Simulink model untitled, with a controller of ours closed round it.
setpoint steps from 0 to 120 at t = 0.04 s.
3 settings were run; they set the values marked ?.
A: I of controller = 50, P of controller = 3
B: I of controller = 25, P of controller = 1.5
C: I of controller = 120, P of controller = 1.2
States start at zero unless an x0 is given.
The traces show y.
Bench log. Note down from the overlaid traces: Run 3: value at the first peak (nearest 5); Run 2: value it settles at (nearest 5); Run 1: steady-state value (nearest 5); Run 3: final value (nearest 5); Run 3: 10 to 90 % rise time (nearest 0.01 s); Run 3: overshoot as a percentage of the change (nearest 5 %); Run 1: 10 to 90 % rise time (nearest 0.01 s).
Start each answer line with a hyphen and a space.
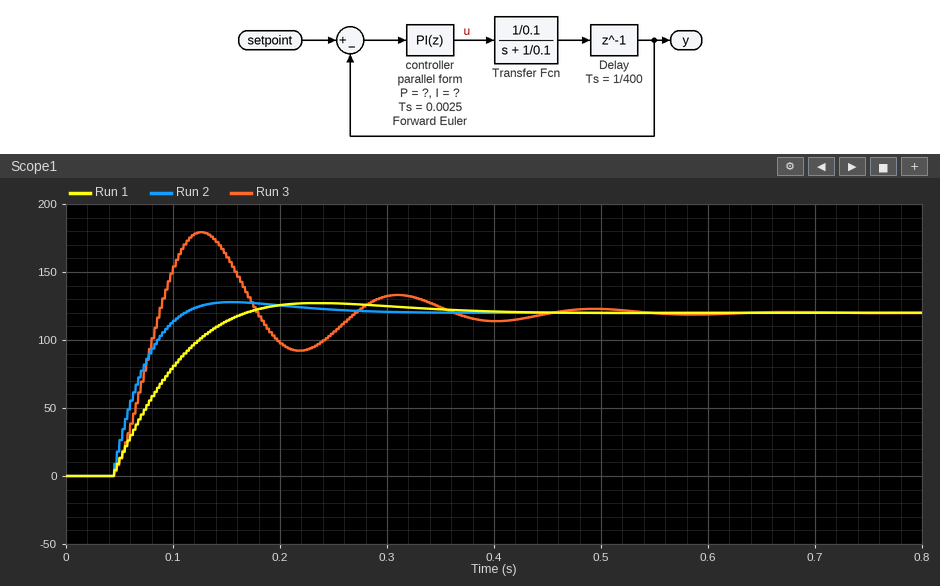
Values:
- 180
- 120
- 120
- 120
- 0.03 s
- 50 %
- 0.09 s
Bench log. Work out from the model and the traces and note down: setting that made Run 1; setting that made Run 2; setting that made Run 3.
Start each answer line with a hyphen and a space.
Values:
- B
- A
- C
